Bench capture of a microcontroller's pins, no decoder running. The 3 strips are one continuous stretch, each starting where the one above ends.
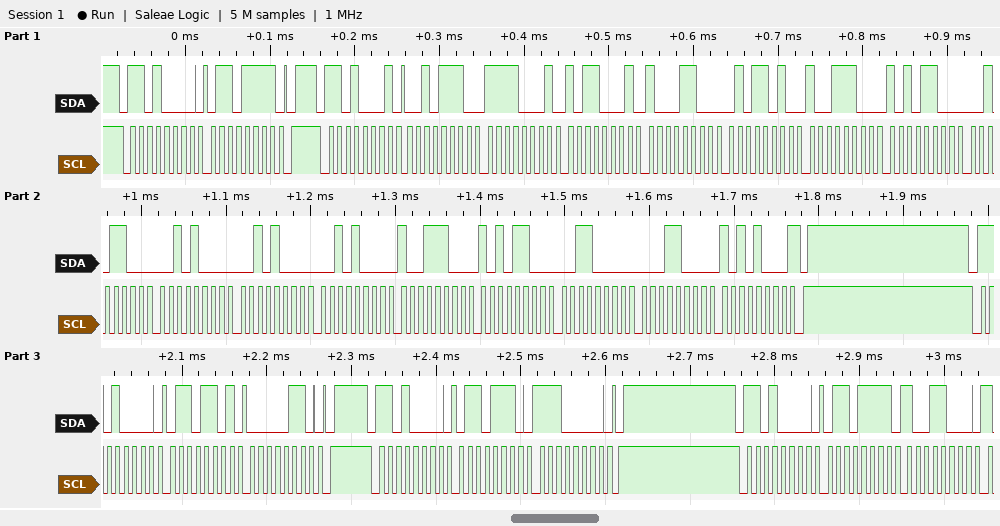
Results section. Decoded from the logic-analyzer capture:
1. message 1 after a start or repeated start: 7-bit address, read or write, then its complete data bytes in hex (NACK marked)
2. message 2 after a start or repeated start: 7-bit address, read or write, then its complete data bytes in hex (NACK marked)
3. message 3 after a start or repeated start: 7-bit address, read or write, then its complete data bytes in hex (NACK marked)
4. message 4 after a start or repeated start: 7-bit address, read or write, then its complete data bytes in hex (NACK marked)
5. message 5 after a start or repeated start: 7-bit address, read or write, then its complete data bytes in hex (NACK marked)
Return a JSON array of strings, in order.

["0x68 write: 6F", "0x68 read: 2E F1 B1 8C 5A 9C AC 2C 28 28 28 9C AC 30 18 A8 NACK", "0x68 write: 6D 06", "0x68 write: 6E E0", "0x68 write: 6F 98"]
